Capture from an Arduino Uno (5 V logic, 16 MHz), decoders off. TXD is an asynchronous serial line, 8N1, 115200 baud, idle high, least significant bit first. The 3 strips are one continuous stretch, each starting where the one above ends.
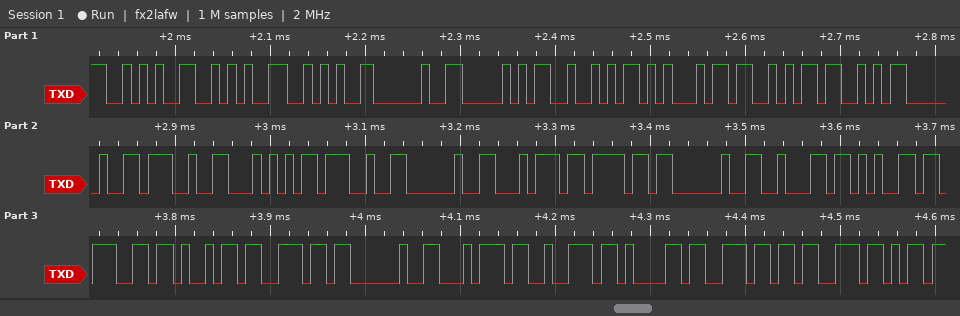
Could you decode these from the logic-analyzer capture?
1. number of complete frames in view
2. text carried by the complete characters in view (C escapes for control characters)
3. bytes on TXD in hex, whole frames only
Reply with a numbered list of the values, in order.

1. 28
2. "*** PRESS 'T' to begin trans"
3. 2A 2A 2A 20 50 52 45 53 53 20 27 54 27 20 74 6F 20 62 65 67 69 6E 20 74 72 61 6E 73
